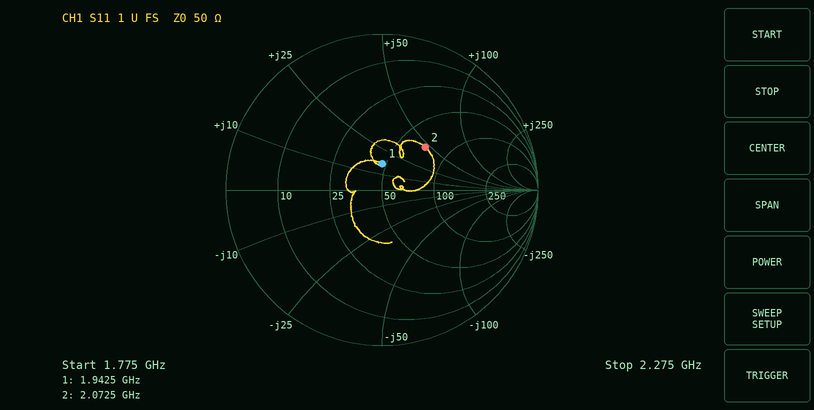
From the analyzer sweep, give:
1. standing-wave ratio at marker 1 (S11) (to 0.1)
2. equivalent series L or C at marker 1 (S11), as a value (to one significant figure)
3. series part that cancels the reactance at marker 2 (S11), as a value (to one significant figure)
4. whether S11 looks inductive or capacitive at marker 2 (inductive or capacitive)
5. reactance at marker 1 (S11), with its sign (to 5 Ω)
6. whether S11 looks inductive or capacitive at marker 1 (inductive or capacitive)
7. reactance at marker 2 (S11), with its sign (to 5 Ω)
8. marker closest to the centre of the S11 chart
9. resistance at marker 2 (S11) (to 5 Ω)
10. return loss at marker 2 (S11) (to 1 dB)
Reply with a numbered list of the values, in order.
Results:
1. 1.4
2. 1 nH
3. 2 pF
4. inductive
5. +15 Ω
6. inductive
7. +45 Ω
8. marker 1
9. 70 Ω
10. 8 dB
